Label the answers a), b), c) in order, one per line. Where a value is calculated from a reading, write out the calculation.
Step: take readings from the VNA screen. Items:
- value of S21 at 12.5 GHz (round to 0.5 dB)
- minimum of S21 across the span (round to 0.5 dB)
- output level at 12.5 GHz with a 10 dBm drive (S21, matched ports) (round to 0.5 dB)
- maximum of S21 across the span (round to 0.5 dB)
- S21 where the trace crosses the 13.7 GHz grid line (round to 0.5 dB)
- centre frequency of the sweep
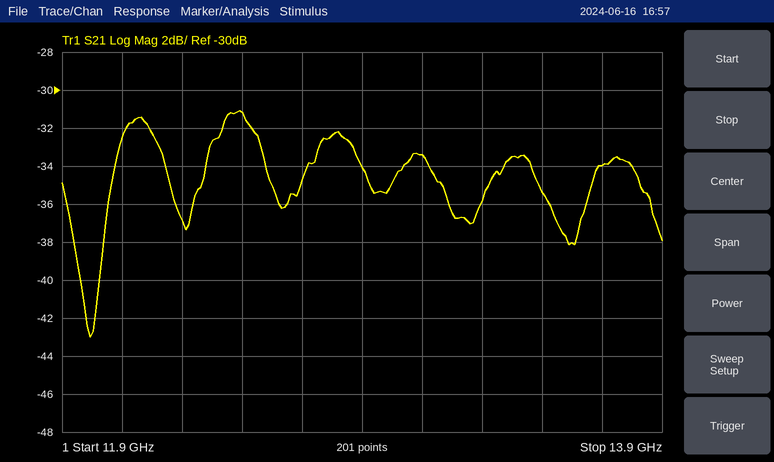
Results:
a) -31.0 dB
b) -43.0 dB
c) 10 dBm + (-31.0 dB) = -21.0 dBm
d) -31.0 dB
e) -34.0 dB
f) 12.9 GHz
